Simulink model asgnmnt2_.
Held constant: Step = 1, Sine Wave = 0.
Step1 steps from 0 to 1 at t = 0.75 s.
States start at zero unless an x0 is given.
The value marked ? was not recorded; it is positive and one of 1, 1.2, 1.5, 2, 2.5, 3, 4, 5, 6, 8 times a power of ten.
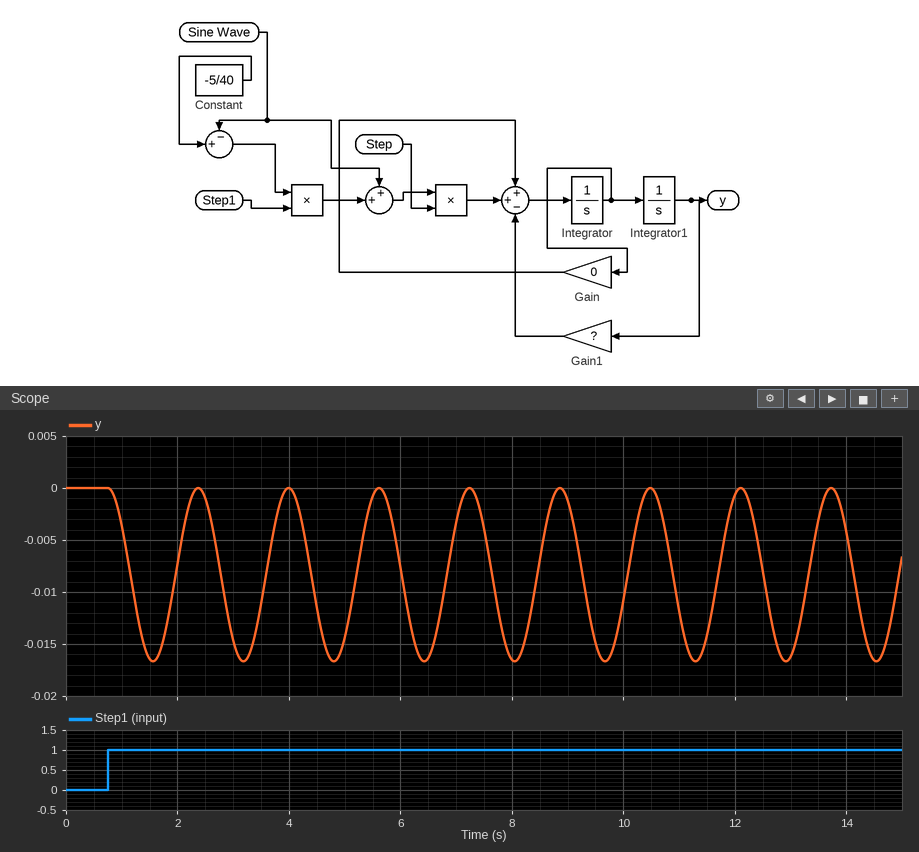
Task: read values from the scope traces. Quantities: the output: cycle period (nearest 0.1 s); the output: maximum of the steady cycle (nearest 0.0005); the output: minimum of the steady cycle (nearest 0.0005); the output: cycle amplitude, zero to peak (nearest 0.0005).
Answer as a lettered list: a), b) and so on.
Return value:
a) 1.6 s
b) 0.0000
c) -0.0165
d) 0.0085
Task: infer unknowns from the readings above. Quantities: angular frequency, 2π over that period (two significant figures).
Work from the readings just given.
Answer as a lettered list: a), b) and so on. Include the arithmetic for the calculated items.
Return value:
a) 2π / 1.6 = 3.9 rad/s
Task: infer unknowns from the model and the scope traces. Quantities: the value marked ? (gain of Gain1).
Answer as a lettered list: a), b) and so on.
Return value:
a) 15
